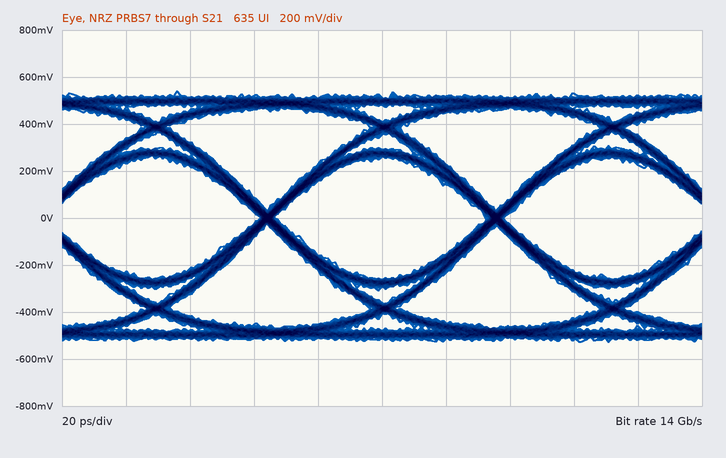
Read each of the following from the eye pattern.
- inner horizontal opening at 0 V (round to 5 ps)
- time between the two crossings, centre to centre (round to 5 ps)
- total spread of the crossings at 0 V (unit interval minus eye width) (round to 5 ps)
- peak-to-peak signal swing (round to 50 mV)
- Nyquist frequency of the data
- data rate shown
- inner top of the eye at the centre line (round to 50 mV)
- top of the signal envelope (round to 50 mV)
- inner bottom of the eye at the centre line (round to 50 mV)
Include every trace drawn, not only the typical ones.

65 ps
70 ps
5 ps
1.05 V
7 GHz
14 Gb/s
250 mV
550 mV
-250 mV
